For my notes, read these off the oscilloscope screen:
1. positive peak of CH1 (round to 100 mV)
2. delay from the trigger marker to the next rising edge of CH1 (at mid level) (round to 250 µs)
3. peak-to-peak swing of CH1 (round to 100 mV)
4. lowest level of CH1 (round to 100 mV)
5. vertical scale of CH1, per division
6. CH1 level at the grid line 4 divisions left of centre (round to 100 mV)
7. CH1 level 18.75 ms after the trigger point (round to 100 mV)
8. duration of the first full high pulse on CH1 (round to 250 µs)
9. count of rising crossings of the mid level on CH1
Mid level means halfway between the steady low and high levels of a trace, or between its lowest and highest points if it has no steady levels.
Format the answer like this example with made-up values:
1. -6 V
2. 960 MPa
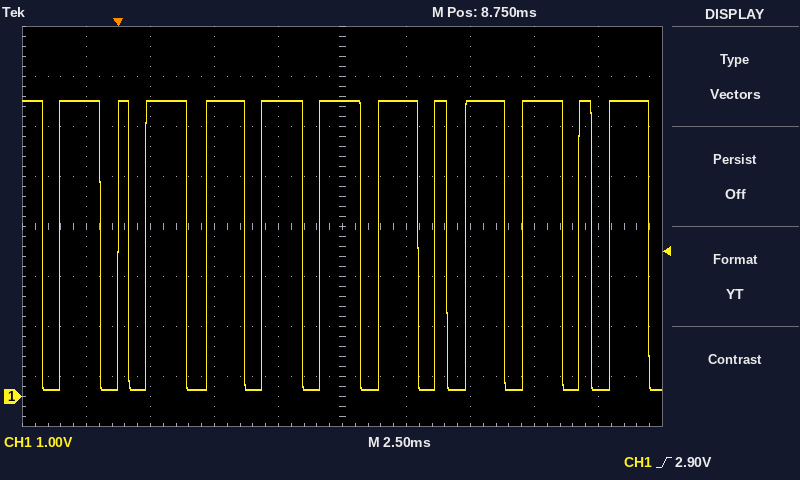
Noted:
1. 5.9 V
2. 1.00 ms
3. 5.8 V
4. 100 mV
5. 1 V
6. 5.9 V
7. 100 mV
8. 1.50 ms
9. 12
